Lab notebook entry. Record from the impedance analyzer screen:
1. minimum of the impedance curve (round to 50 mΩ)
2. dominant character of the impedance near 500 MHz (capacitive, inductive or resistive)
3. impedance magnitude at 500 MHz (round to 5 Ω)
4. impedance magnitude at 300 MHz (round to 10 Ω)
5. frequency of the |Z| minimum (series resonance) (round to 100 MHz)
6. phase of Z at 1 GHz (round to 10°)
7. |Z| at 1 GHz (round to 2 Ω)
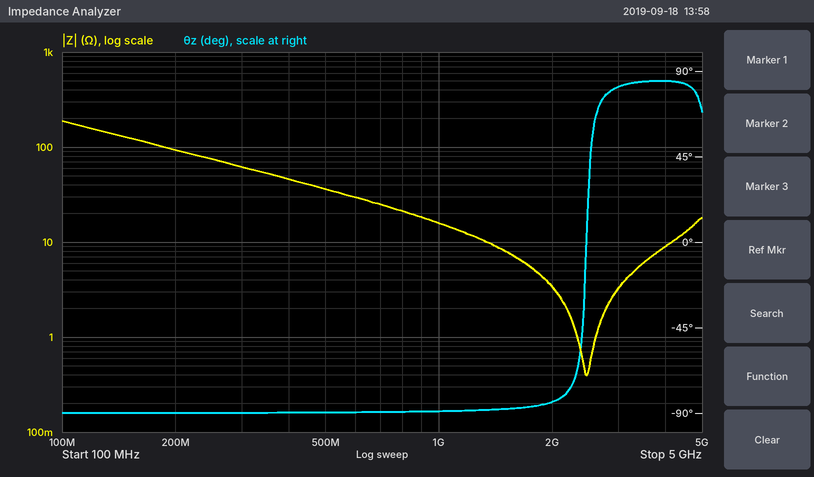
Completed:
400 mΩ
capacitive
35 Ω
60 Ω
2.5 GHz
-90°
16 Ω
